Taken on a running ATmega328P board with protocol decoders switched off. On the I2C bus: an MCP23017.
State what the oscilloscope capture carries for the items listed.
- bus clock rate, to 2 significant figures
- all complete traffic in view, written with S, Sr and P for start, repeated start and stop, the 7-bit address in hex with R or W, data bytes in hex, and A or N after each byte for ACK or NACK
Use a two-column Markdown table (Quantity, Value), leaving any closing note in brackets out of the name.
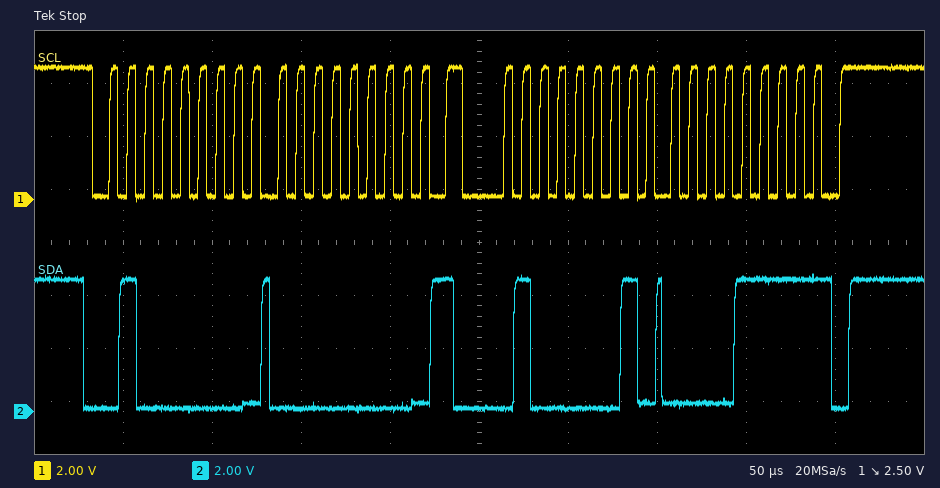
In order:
| Quantity | Value |
|---|---|
| bus clock rate, to 2 significant figures | 100 kHz |
| all complete traffic in view, written with S, Sr and P for start, repeated start and stop, the 7-bit address in hex with R or W, data bytes in hex, and A or N after each byte for ACK or NACK | S 20W A 00 A Sr 20R A 0F N P |
